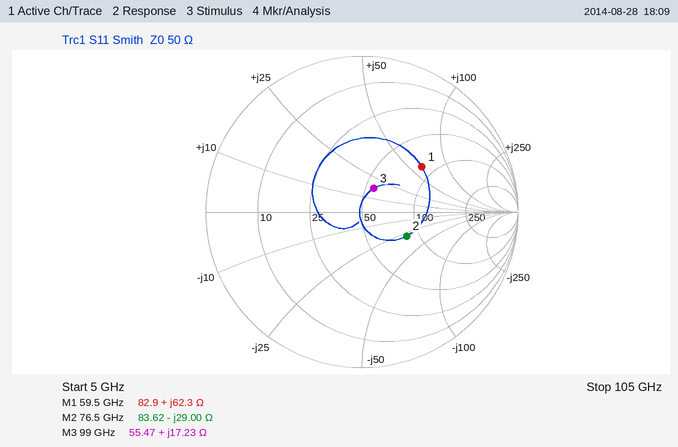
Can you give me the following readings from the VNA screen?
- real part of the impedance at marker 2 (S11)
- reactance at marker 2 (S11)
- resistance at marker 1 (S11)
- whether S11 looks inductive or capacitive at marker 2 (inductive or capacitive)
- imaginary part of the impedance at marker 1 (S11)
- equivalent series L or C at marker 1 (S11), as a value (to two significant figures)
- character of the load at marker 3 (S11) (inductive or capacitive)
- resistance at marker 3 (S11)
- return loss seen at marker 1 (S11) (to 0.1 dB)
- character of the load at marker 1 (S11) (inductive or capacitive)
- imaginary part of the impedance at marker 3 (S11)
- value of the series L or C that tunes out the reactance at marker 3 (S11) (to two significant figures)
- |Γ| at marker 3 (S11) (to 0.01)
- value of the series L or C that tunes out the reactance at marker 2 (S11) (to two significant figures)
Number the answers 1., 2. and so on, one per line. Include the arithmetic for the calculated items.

1. 83.62 Ω
2. -29.00 Ω
3. 82.9 Ω
4. capacitive
5. +62.3 Ω
6. L = 62.3 Ω/(2π × 59.5 GHz) ≈ 167 pH, so 170 pH to two significant figures
7. inductive
8. 55.47 Ω
9. 6.4 dB
10. inductive
11. +17.23 Ω
12. C = 1/(2π × 99 GHz × 17.23 Ω) ≈ 93 fF
13. 0.17
14. L = 29 Ω/(2π × 76.5 GHz) ≈ 60 pH
